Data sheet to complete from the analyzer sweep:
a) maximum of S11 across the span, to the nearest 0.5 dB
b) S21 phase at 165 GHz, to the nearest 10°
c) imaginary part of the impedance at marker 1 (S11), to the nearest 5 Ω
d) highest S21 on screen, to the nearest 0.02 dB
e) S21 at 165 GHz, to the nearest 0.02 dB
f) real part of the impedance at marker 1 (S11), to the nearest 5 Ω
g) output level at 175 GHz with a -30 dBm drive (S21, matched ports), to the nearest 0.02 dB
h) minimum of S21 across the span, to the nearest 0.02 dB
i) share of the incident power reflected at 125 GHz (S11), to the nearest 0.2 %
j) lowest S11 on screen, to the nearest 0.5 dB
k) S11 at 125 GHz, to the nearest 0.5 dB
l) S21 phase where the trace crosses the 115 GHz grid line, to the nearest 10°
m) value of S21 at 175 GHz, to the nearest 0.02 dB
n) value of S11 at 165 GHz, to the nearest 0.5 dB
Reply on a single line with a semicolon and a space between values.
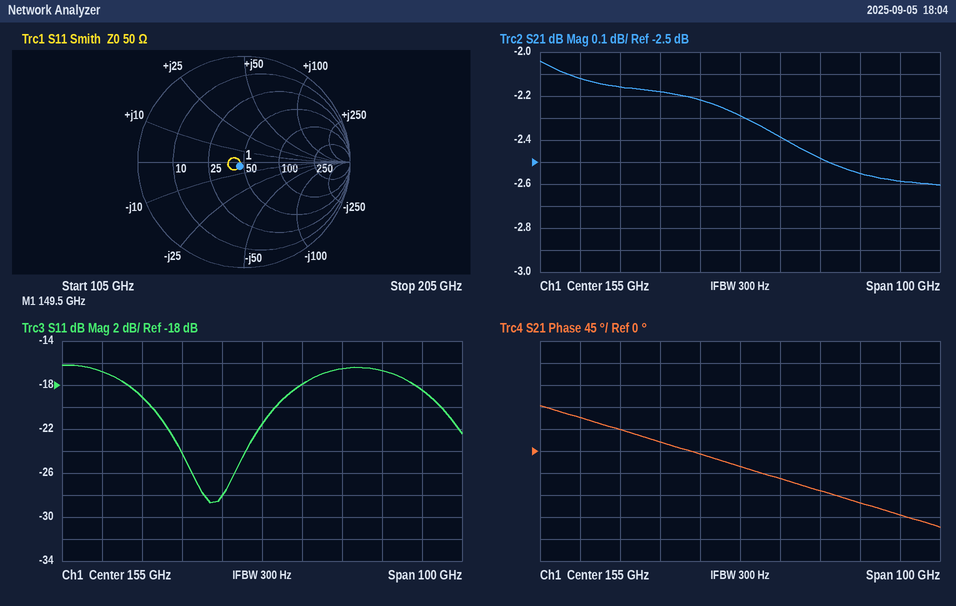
-16.0 dB; -60°; -5 Ω; -2.04 dB; -2.38 dB; 45 Ω; -32.48 dBm; -2.60 dB; 1.2 %; -28.5 dB; -19.0 dB; 70°; -2.48 dB; -18.0 dB
